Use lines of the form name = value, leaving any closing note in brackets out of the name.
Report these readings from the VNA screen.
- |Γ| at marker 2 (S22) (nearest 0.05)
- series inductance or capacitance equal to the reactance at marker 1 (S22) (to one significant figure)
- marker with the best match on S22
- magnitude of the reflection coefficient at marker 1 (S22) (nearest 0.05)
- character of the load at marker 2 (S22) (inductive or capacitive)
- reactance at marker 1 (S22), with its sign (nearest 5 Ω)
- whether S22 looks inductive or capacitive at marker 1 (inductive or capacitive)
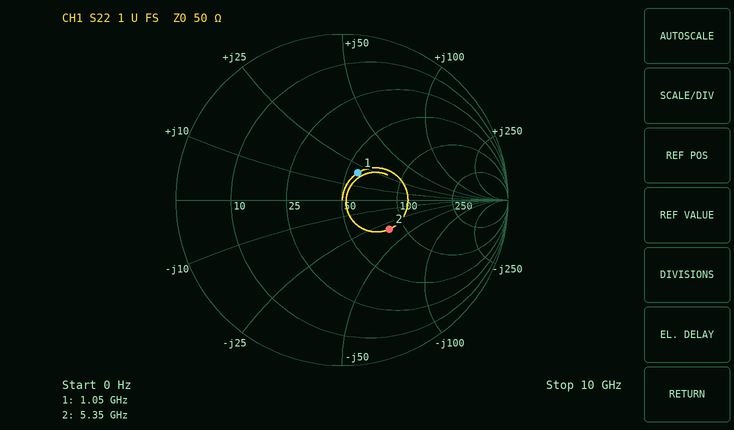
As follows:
|Γ| at marker 2 (S22) = 0.35
series inductance or capacitance equal to the reactance at marker 1 (S22) = 3 nH
marker with the best match on S22 = marker 1
magnitude of the reflection coefficient at marker 1 (S22) = 0.20
character of the load at marker 2 (S22) = capacitive
reactance at marker 1 (S22), with its sign = +20 Ω
whether S22 looks inductive or capacitive at marker 1 = inductive
